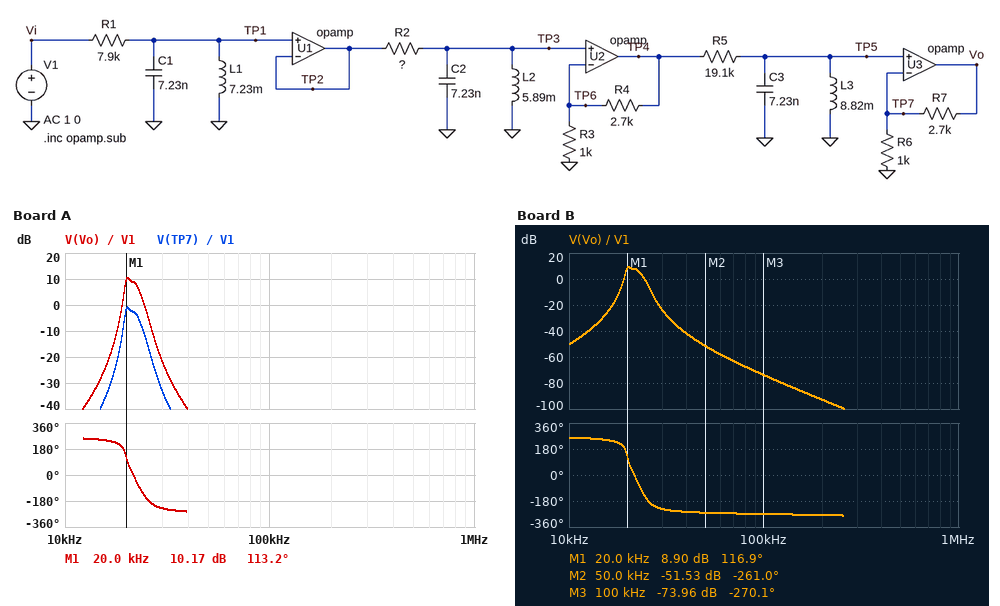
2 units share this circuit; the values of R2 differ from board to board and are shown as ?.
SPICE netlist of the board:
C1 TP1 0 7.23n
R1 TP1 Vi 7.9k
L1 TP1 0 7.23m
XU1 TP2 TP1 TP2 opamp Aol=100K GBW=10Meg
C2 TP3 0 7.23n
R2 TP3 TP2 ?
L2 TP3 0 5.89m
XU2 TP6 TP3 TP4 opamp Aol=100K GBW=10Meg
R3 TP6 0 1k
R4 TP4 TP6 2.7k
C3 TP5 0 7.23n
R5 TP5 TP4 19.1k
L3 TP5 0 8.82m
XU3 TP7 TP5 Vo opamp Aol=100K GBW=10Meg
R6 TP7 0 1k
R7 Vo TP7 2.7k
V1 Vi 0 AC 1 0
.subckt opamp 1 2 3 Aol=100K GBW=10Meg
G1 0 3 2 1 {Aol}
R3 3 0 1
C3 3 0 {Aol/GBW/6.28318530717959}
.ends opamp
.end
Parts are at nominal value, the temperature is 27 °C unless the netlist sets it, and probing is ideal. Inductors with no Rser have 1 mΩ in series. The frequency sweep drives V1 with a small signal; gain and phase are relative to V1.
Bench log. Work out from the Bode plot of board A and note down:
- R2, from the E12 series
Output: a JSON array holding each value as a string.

["4.7 kΩ"]
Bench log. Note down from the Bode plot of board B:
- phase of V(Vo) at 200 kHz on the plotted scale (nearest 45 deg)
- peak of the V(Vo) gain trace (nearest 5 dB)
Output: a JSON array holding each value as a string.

["-270 deg", "10 dB"]
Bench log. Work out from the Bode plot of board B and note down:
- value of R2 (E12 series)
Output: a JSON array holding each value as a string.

["5.6 kΩ"]
